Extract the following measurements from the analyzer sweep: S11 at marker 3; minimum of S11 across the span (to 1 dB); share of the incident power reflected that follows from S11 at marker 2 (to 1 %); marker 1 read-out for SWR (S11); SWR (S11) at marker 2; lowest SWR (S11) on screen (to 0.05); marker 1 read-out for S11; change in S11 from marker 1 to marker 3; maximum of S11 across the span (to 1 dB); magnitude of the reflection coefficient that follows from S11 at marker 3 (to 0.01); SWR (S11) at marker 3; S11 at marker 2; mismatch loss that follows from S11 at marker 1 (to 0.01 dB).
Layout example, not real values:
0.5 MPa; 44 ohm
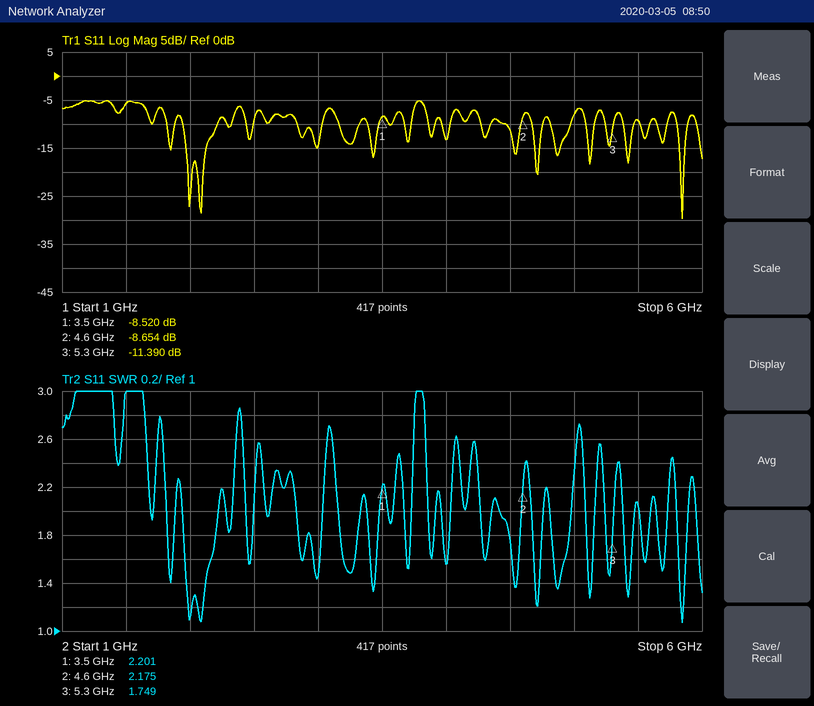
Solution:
-11.390 dB; -30 dB; 14 %; 2.201; 2.175; 1.05; -8.520 dB; -2.870 dB; -5 dB; 0.27; 1.749; -8.654 dB; 0.66 dB
